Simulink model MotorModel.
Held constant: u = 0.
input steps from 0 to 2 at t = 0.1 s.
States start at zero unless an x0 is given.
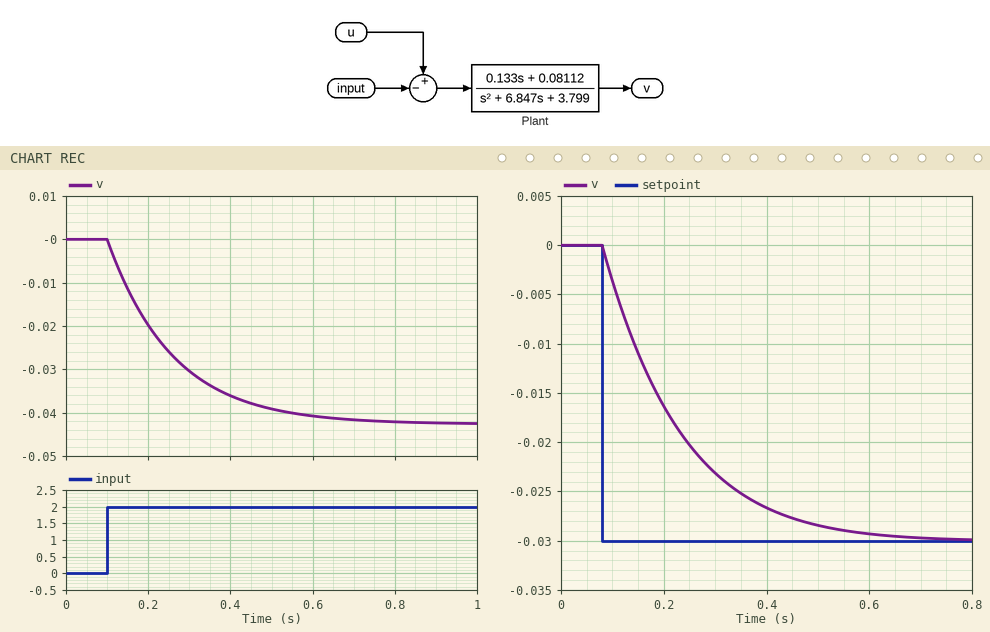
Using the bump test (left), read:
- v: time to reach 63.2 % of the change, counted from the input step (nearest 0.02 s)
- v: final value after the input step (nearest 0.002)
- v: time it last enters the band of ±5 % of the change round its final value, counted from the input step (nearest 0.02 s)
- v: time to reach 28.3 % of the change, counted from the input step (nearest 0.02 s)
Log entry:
0.16 s
-0.042
0.48 s
0.06 s
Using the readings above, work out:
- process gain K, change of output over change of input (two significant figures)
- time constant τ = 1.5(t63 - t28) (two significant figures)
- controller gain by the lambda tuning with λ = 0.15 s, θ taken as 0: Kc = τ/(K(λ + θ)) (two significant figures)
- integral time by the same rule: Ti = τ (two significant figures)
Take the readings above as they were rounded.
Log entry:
-0.021
0.15 s
-48
0.15 s
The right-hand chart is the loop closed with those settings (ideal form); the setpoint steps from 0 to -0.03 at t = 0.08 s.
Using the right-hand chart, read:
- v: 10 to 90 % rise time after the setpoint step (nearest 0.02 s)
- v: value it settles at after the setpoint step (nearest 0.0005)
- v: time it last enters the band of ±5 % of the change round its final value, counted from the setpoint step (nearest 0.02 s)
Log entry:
0.32 s
-0.0300
0.42 s
